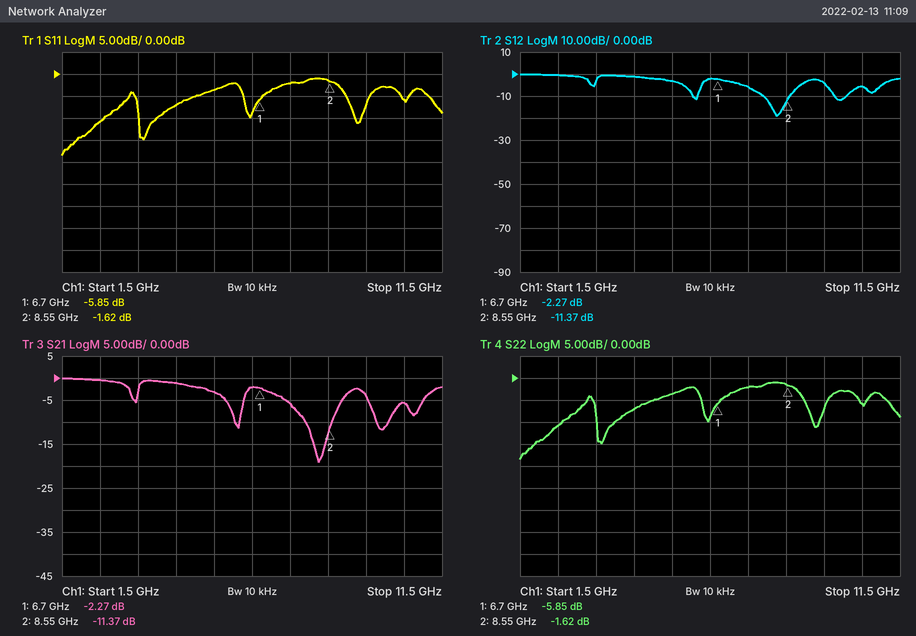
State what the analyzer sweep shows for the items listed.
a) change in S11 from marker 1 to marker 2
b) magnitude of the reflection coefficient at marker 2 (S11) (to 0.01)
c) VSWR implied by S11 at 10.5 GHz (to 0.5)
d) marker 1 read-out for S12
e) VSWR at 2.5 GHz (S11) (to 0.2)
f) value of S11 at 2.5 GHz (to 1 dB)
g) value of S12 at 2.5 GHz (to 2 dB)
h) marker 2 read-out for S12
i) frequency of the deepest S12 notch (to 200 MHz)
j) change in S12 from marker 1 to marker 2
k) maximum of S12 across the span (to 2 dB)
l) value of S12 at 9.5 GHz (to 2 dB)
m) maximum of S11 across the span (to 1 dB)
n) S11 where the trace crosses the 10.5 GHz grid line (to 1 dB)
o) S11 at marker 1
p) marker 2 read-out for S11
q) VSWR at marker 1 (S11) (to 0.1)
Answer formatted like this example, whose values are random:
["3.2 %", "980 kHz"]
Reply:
["4.23 dB", "0.83", "3.0", "-2.27 dB", "1.8", "-11 dB", "0 dB", "-11.37 dB", "8.2 GHz", "-9.10 dB", "0 dB", "-4 dB", "-1 dB", "-6 dB", "-5.85 dB", "-1.62 dB", "3.1"]
